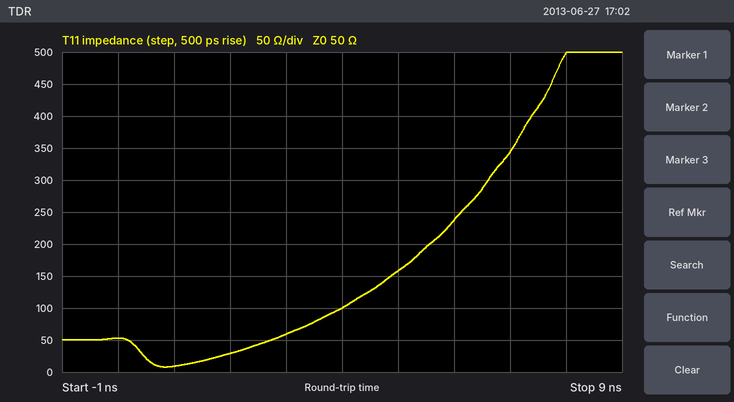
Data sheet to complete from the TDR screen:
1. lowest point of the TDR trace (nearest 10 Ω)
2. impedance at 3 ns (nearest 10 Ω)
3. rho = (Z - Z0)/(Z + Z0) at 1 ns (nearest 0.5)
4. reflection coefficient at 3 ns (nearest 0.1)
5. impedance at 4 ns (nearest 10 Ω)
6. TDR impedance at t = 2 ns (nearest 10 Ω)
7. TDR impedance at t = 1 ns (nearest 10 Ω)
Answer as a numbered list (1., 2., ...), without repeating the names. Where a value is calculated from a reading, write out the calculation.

1. 10 Ω
2. 60 Ω
3. (10 − 50)/(10 + 50) ≈ -0.667, so -0.5 to the nearest 0.5
4. (60 − 50)/(60 + 50) ≈ +0.1
5. 100 Ω
6. 30 Ω
7. 10 Ω
